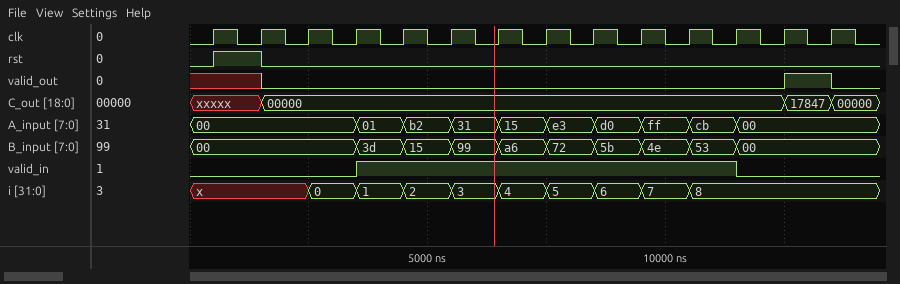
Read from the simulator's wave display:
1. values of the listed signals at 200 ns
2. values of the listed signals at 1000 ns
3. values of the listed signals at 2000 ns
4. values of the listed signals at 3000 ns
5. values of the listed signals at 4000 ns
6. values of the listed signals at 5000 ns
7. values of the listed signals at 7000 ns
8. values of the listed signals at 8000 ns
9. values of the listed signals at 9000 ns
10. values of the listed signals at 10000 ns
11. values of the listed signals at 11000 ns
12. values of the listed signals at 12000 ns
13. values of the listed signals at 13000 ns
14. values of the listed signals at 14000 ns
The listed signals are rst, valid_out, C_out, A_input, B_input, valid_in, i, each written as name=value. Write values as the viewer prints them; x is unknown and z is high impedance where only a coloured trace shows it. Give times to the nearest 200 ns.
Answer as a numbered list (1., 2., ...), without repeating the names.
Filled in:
1. rst=0, valid_out=x, C_out=xxxxx, A_input=00, B_input=00, valid_in=0, i=x
2. rst=1, valid_out=x, C_out=xxxxx, A_input=00, B_input=00, valid_in=0, i=x
3. rst=0, valid_out=0, C_out=00000, A_input=00, B_input=00, valid_in=0, i=x
4. rst=0, valid_out=0, C_out=00000, A_input=00, B_input=00, valid_in=0, i=0
5. rst=0, valid_out=0, C_out=00000, A_input=01, B_input=3d, valid_in=1, i=1
6. rst=0, valid_out=0, C_out=00000, A_input=b2, B_input=15, valid_in=1, i=2
7. rst=0, valid_out=0, C_out=00000, A_input=15, B_input=a6, valid_in=1, i=4
8. rst=0, valid_out=0, C_out=00000, A_input=e3, B_input=72, valid_in=1, i=5
9. rst=0, valid_out=0, C_out=00000, A_input=d0, B_input=5b, valid_in=1, i=6
10. rst=0, valid_out=0, C_out=00000, A_input=ff, B_input=4e, valid_in=1, i=7
11. rst=0, valid_out=0, C_out=00000, A_input=cb, B_input=53, valid_in=1, i=8
12. rst=0, valid_out=0, C_out=00000, A_input=00, B_input=00, valid_in=0, i=8
13. rst=0, valid_out=1, C_out=17847, A_input=00, B_input=00, valid_in=0, i=8
14. rst=0, valid_out=0, C_out=00000, A_input=00, B_input=00, valid_in=0, i=8
